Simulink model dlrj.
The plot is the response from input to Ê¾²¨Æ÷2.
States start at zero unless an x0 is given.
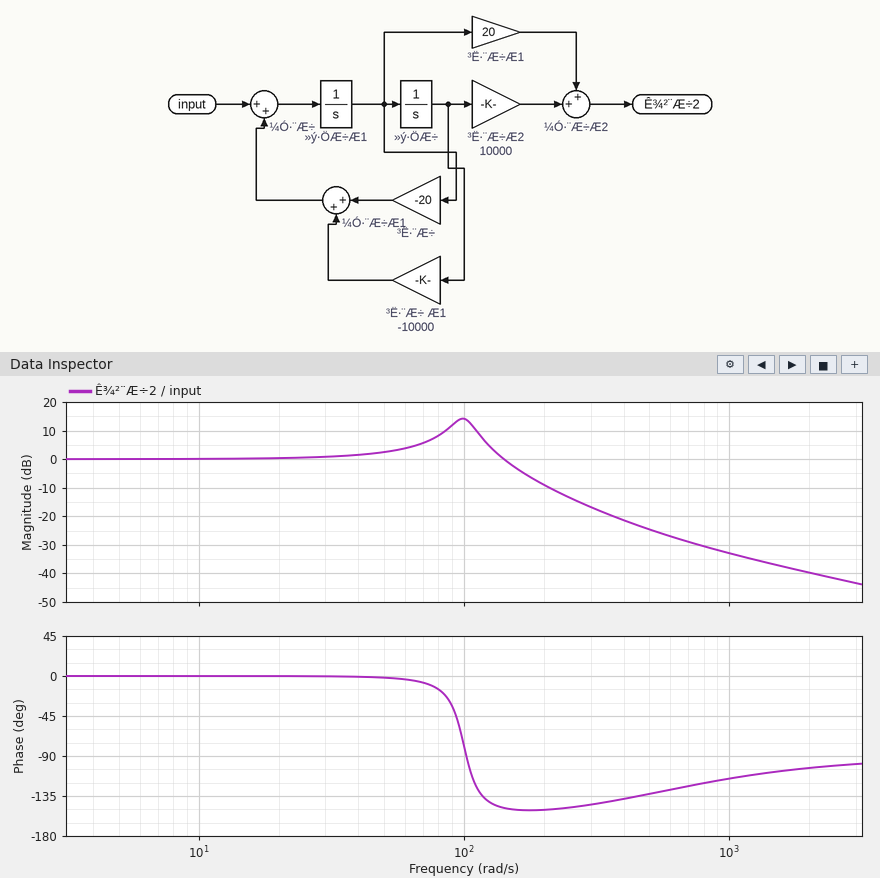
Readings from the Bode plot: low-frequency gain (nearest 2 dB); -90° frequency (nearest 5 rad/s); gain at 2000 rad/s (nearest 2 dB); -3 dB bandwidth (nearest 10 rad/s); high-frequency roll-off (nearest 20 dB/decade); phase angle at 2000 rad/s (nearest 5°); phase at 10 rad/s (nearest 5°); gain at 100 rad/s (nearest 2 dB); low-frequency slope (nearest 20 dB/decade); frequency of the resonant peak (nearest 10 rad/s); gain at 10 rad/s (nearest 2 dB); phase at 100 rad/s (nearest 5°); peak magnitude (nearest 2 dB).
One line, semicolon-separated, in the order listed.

0 dB; 100 rad/s; -40 dB; 160 rad/s; -20 dB/decade; -105°; 0°; 14 dB; 0 dB/decade; 100 rad/s; 0 dB; -80°; 14 dB
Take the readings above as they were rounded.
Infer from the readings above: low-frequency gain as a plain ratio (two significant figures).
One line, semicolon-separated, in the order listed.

1.0
